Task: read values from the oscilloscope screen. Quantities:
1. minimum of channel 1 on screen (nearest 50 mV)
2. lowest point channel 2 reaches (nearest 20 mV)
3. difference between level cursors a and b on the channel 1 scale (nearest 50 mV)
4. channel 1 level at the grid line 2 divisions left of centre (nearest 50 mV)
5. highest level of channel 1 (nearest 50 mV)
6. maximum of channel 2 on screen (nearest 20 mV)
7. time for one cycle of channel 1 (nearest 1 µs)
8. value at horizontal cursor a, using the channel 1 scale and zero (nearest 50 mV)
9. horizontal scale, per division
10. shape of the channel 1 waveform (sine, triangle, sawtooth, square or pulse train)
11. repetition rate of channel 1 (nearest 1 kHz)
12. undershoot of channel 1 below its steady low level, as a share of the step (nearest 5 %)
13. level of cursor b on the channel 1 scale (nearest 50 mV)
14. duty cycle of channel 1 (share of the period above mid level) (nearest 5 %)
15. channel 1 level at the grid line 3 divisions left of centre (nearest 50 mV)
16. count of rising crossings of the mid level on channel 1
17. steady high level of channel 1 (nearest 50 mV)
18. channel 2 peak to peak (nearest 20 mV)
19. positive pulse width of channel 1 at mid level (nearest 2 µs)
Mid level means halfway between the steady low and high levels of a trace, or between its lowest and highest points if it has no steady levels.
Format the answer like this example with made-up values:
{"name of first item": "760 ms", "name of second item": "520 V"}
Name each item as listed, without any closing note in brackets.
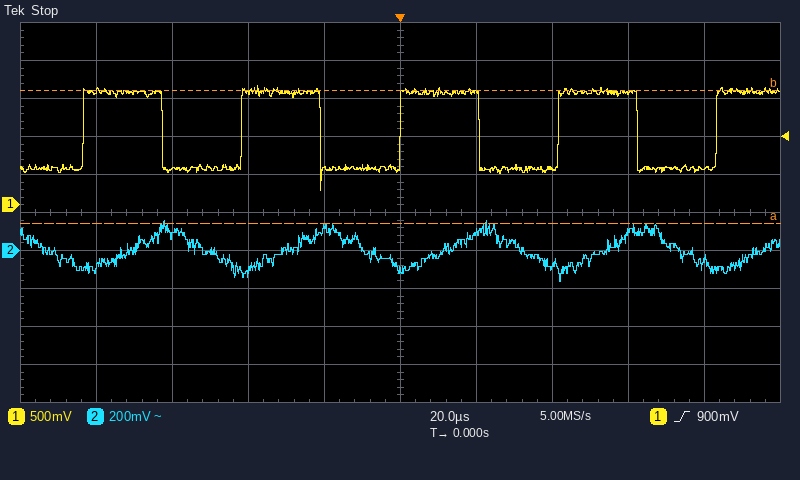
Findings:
{"minimum of channel 1 on screen": "200 mV", "lowest point channel 2 reaches": "-160 mV", "difference between level cursors a and b on the channel 1 scale": "1.75 V", "channel 1 level at the grid line 2 divisions left of centre": "1.50 V", "highest level of channel 1": "1.55 V", "maximum of channel 2 on screen": "160 mV", "time for one cycle of channel 1": "42 µs", "value at horizontal cursor a, using the channel 1 scale and zero": "-250 mV", "horizontal scale, per division": "20 µs", "shape of the channel 1 waveform": "square", "repetition rate of channel 1": "24 kHz", "undershoot of channel 1 below its steady low level, as a share of the step": "30 %", "level of cursor b on the channel 1 scale": "1.50 V", "duty cycle of channel 1 (share of the period above mid level)": "50 %", "channel 1 level at the grid line 3 divisions left of centre": "450 mV", "count of rising crossings of the mid level on channel 1": "5", "steady high level of channel 1": "1.50 V", "channel 2 peak to peak": "320 mV", "positive pulse width of channel 1 at mid level": "20 µs"}
